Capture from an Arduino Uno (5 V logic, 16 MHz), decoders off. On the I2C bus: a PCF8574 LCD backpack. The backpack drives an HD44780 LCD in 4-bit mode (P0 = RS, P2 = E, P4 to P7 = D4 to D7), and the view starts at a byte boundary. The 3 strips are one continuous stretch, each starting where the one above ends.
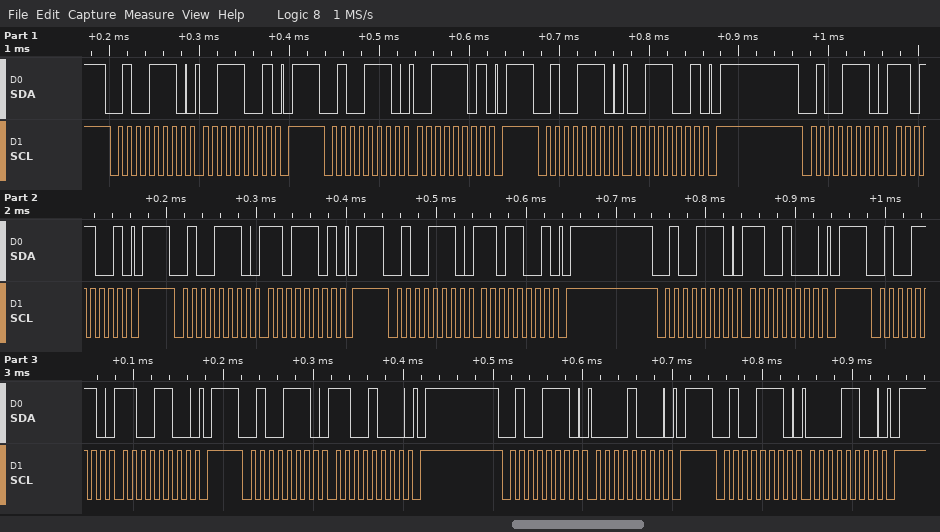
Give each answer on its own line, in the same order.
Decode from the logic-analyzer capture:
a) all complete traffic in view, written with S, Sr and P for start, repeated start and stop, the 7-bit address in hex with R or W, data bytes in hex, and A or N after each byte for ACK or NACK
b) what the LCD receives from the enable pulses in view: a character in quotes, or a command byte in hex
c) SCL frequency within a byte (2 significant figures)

S 27W A 39 A P S 27W A 3D A P S 27W A 39 A P S 27W A D9 A P S 27W A DD A P S 27W A D9 A P S 27W A C8 A P S 27W A CC A P S 27W A C8 A P S 27W A 08 A P S 27W A 0C A P
'='
100 kHz
